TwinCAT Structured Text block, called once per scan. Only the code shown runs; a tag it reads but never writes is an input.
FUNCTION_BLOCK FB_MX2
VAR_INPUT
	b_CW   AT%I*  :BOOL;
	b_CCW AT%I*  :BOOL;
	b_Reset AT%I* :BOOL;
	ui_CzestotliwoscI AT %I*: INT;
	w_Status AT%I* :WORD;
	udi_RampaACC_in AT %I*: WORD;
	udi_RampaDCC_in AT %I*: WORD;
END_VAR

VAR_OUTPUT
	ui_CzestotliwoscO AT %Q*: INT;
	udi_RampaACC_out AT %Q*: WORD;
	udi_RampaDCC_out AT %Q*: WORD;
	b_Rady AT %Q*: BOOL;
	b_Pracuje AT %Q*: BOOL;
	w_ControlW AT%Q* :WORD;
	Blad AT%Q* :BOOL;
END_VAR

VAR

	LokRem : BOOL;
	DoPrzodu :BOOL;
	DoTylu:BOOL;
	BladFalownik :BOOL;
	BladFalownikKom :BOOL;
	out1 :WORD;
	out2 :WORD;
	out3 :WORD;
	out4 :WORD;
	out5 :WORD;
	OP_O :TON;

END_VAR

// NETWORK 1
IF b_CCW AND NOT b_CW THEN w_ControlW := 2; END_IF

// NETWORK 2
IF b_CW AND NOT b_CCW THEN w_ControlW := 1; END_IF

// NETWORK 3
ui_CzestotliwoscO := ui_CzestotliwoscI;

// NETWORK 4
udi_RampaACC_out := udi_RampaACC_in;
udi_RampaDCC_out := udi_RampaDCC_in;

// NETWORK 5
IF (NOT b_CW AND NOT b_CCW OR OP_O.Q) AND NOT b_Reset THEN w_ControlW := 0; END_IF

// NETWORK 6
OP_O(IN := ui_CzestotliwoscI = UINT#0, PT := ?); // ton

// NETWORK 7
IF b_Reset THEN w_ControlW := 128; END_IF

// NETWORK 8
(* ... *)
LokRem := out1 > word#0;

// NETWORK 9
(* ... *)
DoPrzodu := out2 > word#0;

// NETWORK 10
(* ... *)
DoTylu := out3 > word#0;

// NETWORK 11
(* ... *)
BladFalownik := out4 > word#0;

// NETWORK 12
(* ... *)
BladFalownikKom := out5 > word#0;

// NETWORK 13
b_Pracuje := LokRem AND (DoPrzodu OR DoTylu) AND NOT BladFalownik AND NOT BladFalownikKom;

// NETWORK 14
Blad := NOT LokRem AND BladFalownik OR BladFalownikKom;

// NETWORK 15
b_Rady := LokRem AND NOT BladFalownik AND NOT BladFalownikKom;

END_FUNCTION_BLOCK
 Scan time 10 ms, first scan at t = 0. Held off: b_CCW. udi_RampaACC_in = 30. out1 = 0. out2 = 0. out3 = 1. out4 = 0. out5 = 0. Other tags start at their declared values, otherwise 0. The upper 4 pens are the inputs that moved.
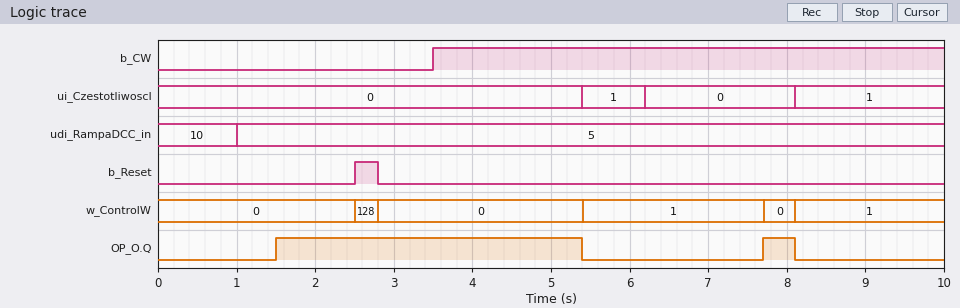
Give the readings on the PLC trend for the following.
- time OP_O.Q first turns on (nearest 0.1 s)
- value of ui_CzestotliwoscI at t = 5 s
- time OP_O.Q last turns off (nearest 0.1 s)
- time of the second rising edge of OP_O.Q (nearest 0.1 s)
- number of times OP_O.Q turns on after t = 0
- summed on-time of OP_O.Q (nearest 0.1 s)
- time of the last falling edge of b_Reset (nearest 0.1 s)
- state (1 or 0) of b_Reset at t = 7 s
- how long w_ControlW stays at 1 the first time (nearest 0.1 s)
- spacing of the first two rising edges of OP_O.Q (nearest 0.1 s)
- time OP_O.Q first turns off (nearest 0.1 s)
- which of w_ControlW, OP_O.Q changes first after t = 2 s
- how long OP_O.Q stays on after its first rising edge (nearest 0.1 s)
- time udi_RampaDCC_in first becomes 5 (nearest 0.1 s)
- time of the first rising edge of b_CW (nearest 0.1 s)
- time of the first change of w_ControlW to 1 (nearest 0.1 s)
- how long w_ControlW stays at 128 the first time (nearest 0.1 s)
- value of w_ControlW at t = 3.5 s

1.5 s
0
8.1 s
7.7 s
2
4.3 s
2.8 s
0
2.3 s
6.2 s
5.4 s
w_ControlW
3.9 s
1.0 s
3.5 s
5.4 s
0.3 s
0
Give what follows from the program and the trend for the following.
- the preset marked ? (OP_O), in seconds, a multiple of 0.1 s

1.5 s
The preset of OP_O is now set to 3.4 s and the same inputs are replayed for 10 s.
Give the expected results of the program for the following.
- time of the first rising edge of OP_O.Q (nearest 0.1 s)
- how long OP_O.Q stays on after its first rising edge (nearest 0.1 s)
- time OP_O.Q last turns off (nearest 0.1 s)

3.4 s
2.0 s
5.4 s
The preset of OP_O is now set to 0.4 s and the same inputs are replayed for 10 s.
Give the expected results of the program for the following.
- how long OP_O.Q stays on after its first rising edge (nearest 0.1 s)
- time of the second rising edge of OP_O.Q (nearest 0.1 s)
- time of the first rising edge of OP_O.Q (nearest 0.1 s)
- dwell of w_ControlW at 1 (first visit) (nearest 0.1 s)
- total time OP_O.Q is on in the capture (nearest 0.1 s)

5.0 s
6.6 s
0.4 s
1.2 s
6.5 s
